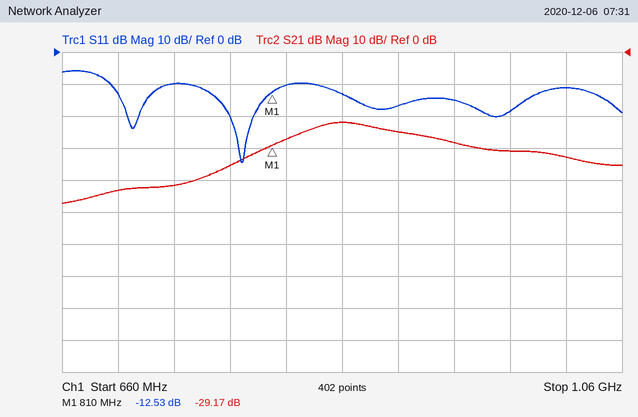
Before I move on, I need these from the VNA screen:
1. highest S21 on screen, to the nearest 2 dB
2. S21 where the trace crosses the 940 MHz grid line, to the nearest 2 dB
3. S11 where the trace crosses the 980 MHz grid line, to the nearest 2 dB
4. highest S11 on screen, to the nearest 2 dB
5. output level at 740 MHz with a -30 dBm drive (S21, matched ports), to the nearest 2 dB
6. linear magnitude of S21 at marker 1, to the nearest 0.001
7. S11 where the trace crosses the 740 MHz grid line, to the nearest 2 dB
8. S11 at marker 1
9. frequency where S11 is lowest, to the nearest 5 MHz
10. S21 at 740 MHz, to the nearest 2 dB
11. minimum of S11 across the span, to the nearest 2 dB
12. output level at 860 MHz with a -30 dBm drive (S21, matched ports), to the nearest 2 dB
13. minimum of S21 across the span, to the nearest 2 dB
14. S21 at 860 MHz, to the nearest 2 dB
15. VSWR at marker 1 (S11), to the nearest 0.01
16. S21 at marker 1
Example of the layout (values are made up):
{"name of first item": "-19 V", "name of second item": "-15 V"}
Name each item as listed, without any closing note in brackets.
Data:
{"highest S21 on screen, to the nearest 2 dB": "-22 dB", "S21 where the trace crosses the 940 MHz grid line, to the nearest 2 dB": "-28 dB", "S11 where the trace crosses the 980 MHz grid line, to the nearest 2 dB": "-18 dB", "highest S11 on screen, to the nearest 2 dB": "-6 dB", "output level at 740 MHz with a -30 dBm drive (S21, matched ports), to the nearest 2 dB": "-72 dBm", "linear magnitude of S21 at marker 1, to the nearest 0.001": "0.035", "S11 where the trace crosses the 740 MHz grid line, to the nearest 2 dB": "-10 dB", "S11 at marker 1": "-12.53 dB", "frequency where S11 is lowest, to the nearest 5 MHz": "790 MHz", "S21 at 740 MHz, to the nearest 2 dB": "-42 dB", "minimum of S11 across the span, to the nearest 2 dB": "-34 dB", "output level at 860 MHz with a -30 dBm drive (S21, matched ports), to the nearest 2 dB": "-52 dBm", "minimum of S21 across the span, to the nearest 2 dB": "-48 dB", "S21 at 860 MHz, to the nearest 2 dB": "-22 dB", "VSWR at marker 1 (S11), to the nearest 0.01": "1.62", "S21 at marker 1": "-29.17 dB"}
